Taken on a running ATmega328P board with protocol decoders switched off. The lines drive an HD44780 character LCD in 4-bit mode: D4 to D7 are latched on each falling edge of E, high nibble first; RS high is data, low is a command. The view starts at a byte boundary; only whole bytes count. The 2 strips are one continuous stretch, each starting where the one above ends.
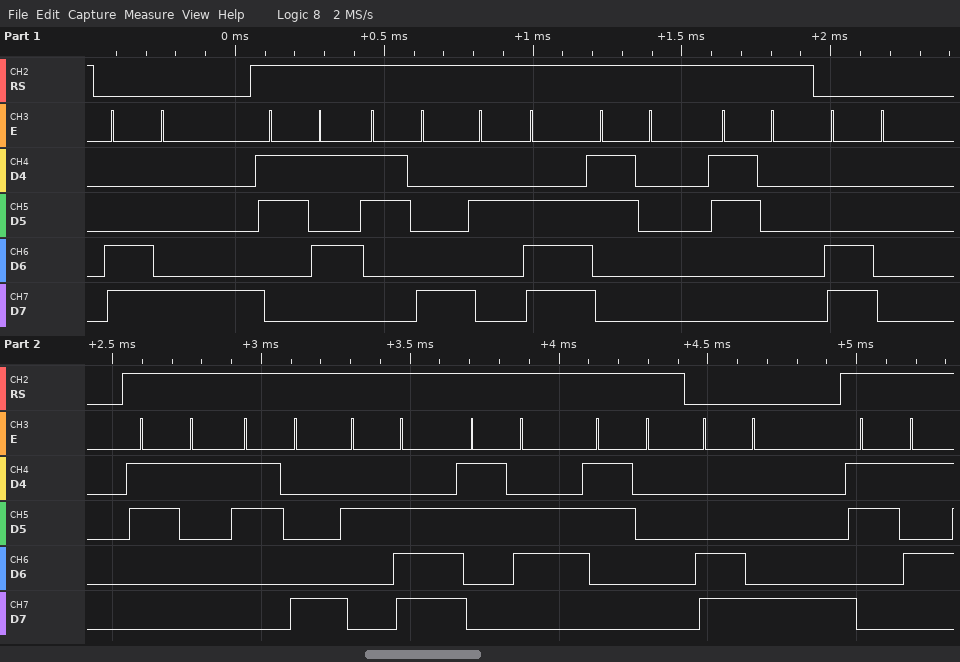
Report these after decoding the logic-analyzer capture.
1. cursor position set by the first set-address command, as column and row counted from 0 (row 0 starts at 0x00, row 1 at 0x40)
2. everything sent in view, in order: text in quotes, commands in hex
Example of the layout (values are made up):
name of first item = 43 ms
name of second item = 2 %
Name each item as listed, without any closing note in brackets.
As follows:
cursor position set by the first set-address command, as column and row counted from 0 = column 8, row 1
everything sent in view, in order: text in quotes, commands in hex = 0xC8 "58.00" 0xC0 "18.60" 0xC8 "5"
